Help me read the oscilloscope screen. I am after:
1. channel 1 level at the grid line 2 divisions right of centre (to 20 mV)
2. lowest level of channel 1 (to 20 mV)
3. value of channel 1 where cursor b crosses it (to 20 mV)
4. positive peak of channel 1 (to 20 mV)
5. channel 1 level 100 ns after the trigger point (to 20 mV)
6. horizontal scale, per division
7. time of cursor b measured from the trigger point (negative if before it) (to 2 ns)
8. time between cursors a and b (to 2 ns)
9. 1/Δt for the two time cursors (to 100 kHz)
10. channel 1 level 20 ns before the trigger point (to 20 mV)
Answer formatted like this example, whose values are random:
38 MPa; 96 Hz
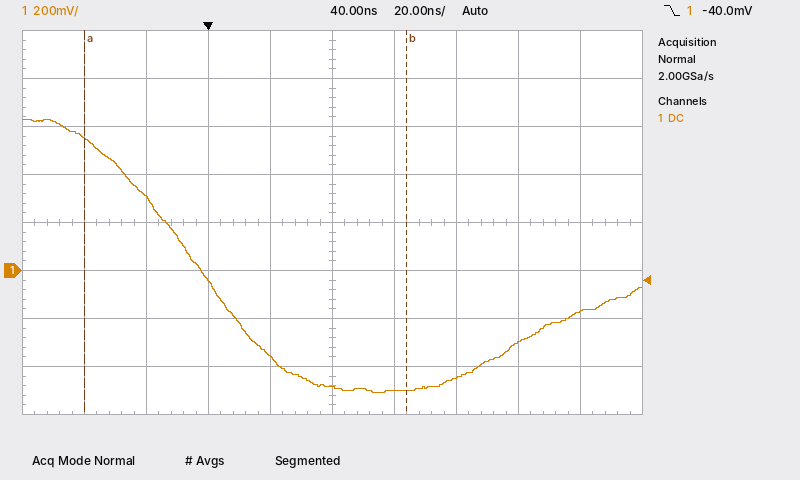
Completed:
-440 mV; -500 mV; -500 mV; 620 mV; -300 mV; 20 ns; +64 ns; 104 ns; 9.6 MHz; 300 mV
